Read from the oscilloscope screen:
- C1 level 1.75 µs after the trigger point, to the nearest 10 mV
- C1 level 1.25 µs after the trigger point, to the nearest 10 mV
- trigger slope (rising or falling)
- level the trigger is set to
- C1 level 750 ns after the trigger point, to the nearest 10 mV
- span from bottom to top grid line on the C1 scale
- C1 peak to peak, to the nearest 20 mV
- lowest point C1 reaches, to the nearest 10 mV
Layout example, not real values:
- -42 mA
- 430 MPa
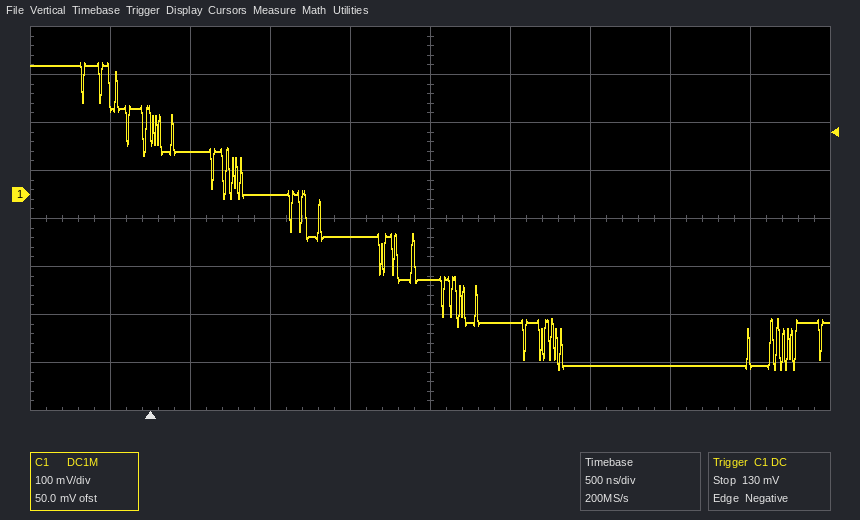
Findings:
- -180 mV
- -90 mV
- falling
- 130 mV
- 0 mV
- 800 mV
- 640 mV
- -360 mV
